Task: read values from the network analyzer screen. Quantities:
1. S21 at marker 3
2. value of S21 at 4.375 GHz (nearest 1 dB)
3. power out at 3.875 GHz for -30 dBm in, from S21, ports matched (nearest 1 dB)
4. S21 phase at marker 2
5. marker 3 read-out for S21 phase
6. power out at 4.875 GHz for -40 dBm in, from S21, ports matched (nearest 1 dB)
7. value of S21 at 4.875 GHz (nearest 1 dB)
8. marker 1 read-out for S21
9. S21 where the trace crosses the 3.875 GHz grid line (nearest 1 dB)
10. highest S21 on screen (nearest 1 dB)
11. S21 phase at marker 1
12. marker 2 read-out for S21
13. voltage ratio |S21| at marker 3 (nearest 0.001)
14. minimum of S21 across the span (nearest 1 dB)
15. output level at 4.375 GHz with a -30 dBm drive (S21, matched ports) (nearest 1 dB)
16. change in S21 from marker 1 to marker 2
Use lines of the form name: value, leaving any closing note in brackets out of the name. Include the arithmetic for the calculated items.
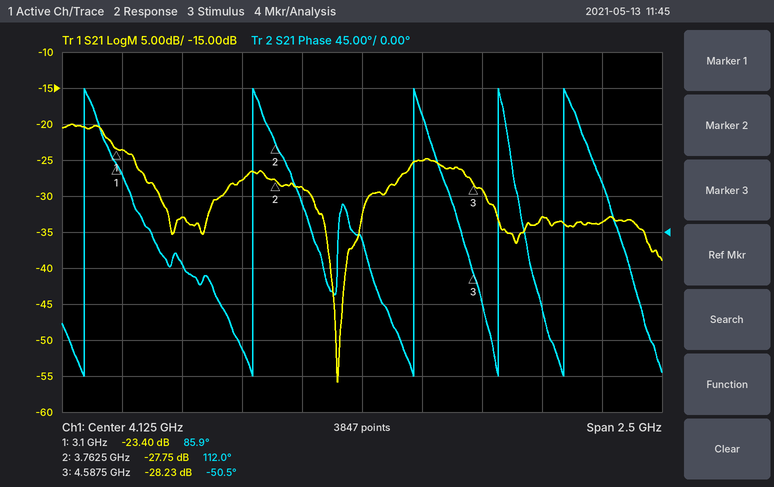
S21 at marker 3: -28.23 dB
value of S21 at 4.375 GHz: -25 dB
power out at 3.875 GHz for -30 dBm in, from S21, ports matched: -30 dBm + (-29 dB) = -59 dBm
S21 phase at marker 2: 112.0°
marker 3 read-out for S21 phase: -50.5°
power out at 4.875 GHz for -40 dBm in, from S21, ports matched: -40 dBm + (-33 dB) = -73 dBm
value of S21 at 4.875 GHz: -33 dB
marker 1 read-out for S21: -23.40 dB
S21 where the trace crosses the 3.875 GHz grid line: -29 dB
highest S21 on screen: -20 dB
S21 phase at marker 1: 85.9°
marker 2 read-out for S21: -27.75 dB
voltage ratio |S21| at marker 3: 10^(-28.23/20) ≈ 0.039
minimum of S21 across the span: -56 dB
output level at 4.375 GHz with a -30 dBm drive (S21, matched ports): -30 dBm + (-25 dB) = -55 dBm
change in S21 from marker 1 to marker 2: -27.75 − (-23.4) = -4.35 dB
